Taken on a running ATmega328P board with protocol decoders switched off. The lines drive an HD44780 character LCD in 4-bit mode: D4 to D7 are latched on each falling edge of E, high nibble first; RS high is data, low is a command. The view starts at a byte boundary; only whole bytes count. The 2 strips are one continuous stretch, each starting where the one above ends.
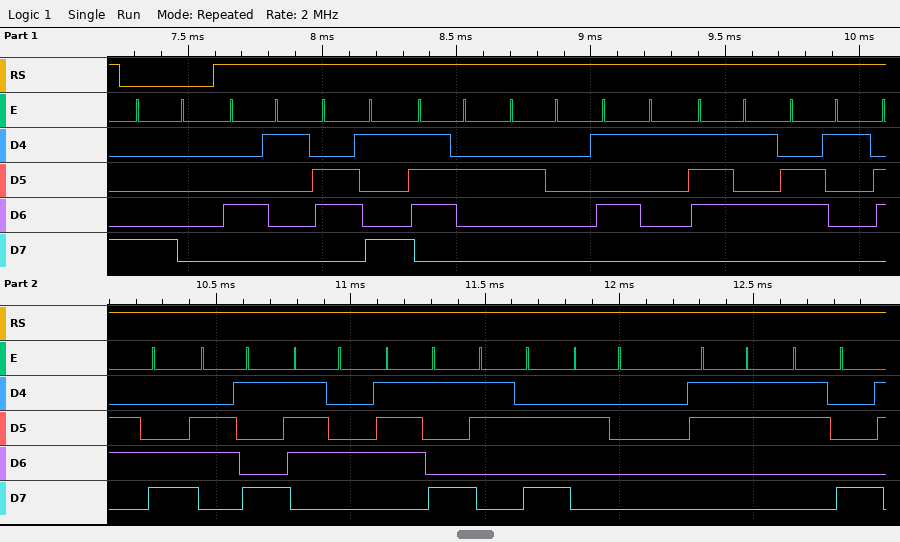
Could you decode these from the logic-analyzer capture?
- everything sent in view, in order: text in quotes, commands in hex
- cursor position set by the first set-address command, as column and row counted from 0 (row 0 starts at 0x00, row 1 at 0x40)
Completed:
0x80 "Air Quality: 38"
column 0, row 0
